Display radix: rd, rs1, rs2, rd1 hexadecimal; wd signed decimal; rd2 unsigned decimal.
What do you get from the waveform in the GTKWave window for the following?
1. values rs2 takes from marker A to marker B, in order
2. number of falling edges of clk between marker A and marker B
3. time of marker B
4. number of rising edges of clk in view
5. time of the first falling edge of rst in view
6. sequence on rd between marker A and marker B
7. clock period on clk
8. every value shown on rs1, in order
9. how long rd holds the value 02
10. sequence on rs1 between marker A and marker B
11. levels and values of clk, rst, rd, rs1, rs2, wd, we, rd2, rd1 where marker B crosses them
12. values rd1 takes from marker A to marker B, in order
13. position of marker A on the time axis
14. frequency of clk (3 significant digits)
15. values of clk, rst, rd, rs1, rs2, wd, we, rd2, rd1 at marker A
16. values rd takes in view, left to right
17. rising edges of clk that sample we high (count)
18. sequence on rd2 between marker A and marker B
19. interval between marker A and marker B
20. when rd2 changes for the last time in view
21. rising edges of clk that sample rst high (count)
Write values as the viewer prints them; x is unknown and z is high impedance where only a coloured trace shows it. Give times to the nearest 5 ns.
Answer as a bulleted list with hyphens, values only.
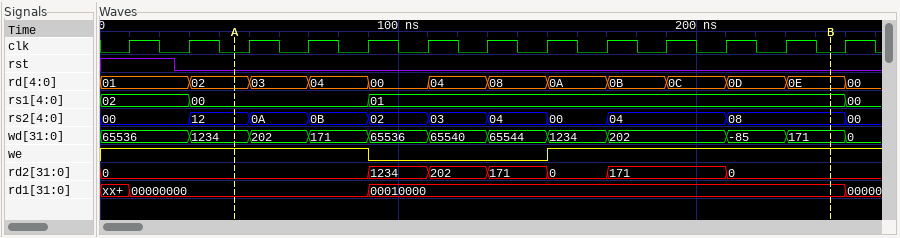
- 12, 0A, 0B, 02, 03, 04, 00, 04, 08
- 10
- 245 ns
- 13
- 25 ns
- 02, 03, 04, 00, 04, 08, 0A, 0B, 0C, 0D, 0E
- 20 ns
- 02, 00, 01, 00
- 20 ns
- 00, 01
- clk=0, rst=0, rd=0E, rs1=01, rs2=08, wd=171, we=1, rd2=0, rd1=00010000
- 00000000, 00010000
- 45 ns
- 50.0 MHz
- clk=0, rst=0, rd=02, rs1=00, rs2=12, wd=1234, we=1, rd2=0, rd1=00000000
- 01, 02, 03, 04, 00, 04, 08, 0A, 0B, 0C, 0D, 0E, 00
- 10
- 0, 1234, 202, 171, 0, 171, 0
- 200 ns
- 210 ns
- 1
